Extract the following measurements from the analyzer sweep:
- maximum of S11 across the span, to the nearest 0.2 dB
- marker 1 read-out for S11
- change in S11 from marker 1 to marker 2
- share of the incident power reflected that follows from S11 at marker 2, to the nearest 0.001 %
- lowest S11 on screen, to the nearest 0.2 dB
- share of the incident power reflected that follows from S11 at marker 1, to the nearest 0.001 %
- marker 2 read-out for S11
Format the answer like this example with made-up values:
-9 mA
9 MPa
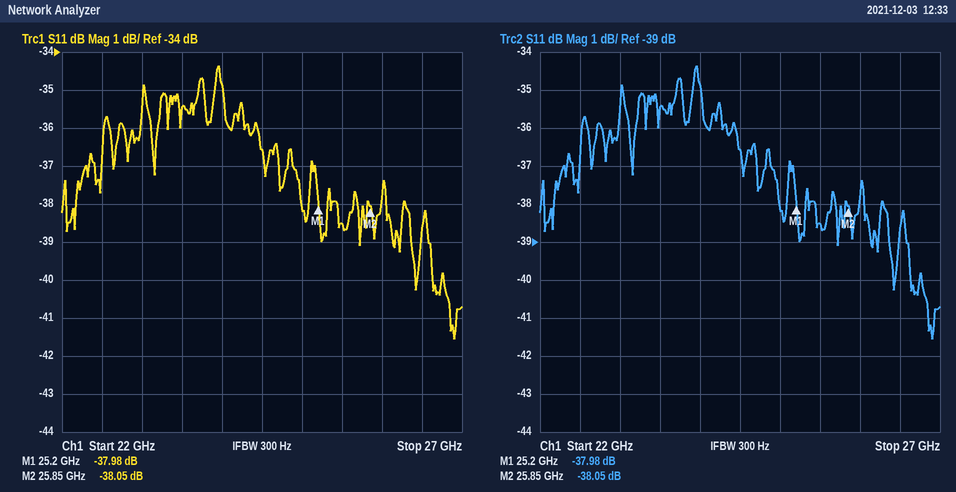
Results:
-34.4 dB
-37.98 dB
-0.07 dB
0.016 %
-41.6 dB
0.016 %
-38.05 dB
